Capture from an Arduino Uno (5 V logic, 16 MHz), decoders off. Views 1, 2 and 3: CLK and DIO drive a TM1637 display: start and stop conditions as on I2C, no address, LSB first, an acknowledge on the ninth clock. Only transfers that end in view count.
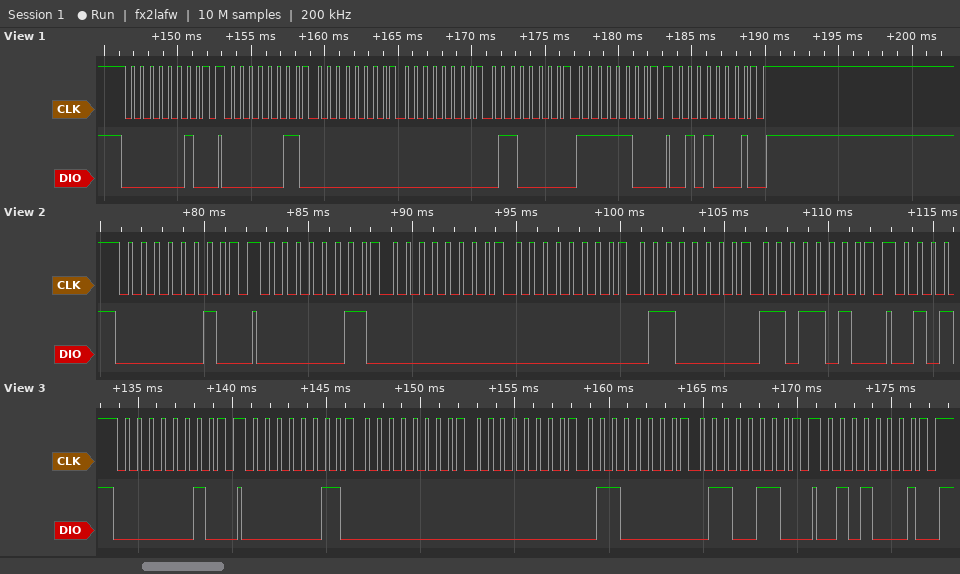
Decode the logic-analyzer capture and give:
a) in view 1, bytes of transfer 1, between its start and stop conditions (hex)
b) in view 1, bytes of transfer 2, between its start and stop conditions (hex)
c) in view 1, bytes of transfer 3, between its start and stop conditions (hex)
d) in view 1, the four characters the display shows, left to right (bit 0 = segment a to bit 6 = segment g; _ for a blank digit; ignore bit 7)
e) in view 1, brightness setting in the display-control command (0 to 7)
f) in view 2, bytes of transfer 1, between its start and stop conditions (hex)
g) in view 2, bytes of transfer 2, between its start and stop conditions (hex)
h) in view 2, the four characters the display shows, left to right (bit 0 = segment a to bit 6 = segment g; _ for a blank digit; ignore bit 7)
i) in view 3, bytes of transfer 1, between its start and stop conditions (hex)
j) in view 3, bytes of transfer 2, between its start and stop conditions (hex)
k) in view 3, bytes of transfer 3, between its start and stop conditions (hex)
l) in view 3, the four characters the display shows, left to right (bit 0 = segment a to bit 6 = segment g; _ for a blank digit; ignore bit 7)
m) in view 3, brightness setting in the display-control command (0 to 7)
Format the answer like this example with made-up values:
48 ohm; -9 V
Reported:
40; C0 00 00 06 3F; 8A; __10; 2; 40; C0 00 00 06 5B; __12; 40; C0 00 00 06 66; 8A; __14; 2
